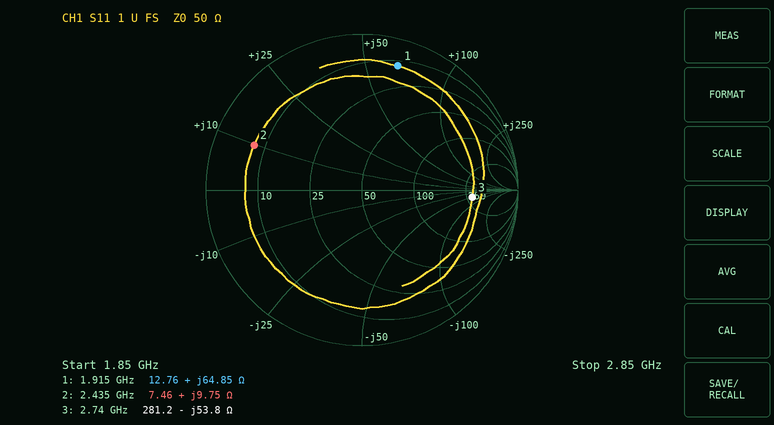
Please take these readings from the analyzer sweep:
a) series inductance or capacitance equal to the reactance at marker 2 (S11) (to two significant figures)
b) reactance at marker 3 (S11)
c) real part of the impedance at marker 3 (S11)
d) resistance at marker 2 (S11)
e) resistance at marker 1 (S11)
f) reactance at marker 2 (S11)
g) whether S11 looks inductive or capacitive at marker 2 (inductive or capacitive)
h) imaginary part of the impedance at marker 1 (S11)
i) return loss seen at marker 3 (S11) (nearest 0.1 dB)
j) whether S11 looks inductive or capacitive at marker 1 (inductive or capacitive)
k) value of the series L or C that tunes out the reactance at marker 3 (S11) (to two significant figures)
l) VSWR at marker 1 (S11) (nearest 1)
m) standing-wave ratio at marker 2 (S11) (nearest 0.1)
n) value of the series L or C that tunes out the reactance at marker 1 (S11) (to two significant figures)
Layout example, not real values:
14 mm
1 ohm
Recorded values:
640 pH
-53.8 Ω
281.2 Ω
7.46 Ω
12.76 Ω
+9.75 Ω
inductive
+64.85 Ω
3.0 dB
inductive
3.1 nH
11
7.0
1.3 pF
